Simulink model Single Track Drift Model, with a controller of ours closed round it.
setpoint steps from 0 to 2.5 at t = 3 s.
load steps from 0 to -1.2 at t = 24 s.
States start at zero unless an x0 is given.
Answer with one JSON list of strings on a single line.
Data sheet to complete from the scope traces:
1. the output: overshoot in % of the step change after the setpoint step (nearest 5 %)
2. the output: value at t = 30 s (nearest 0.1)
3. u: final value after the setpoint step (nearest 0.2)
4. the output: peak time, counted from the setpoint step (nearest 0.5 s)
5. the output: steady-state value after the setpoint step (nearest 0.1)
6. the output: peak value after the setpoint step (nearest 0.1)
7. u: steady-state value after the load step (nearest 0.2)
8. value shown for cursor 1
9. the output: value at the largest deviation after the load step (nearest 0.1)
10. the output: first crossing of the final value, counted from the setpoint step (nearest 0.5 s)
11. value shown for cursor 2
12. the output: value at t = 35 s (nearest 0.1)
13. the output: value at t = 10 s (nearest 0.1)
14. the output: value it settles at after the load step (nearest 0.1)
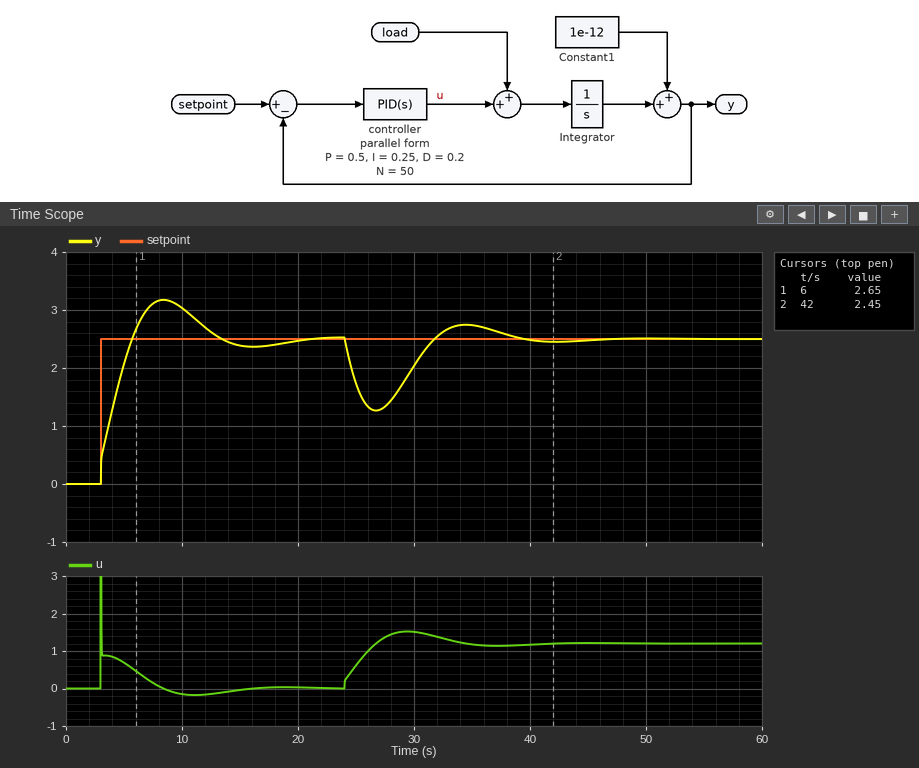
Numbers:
["25 %", "2.0", "0.0", "5.5 s", "2.5", "3.2", "1.2", "2.65", "1.3", "2.5 s", "2.45", "2.7", "3.0", "2.5"]
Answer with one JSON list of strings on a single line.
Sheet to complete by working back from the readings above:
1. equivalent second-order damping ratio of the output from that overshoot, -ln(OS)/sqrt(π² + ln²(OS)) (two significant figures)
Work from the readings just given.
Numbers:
["0.40"]
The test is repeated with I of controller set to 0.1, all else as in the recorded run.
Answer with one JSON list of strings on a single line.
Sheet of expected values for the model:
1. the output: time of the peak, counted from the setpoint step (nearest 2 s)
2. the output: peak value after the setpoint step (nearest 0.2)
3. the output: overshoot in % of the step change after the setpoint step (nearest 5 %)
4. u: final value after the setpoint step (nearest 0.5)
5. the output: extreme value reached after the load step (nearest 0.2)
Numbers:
["8 s", "3.0", "15 %", "0.0", "1.0"]
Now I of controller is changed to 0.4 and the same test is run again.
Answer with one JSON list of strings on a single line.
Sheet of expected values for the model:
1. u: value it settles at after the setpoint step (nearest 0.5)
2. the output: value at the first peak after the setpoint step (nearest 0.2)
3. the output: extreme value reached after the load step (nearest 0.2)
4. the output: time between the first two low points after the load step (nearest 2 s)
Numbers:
["0.0", "3.4", "1.4", "12 s"]
